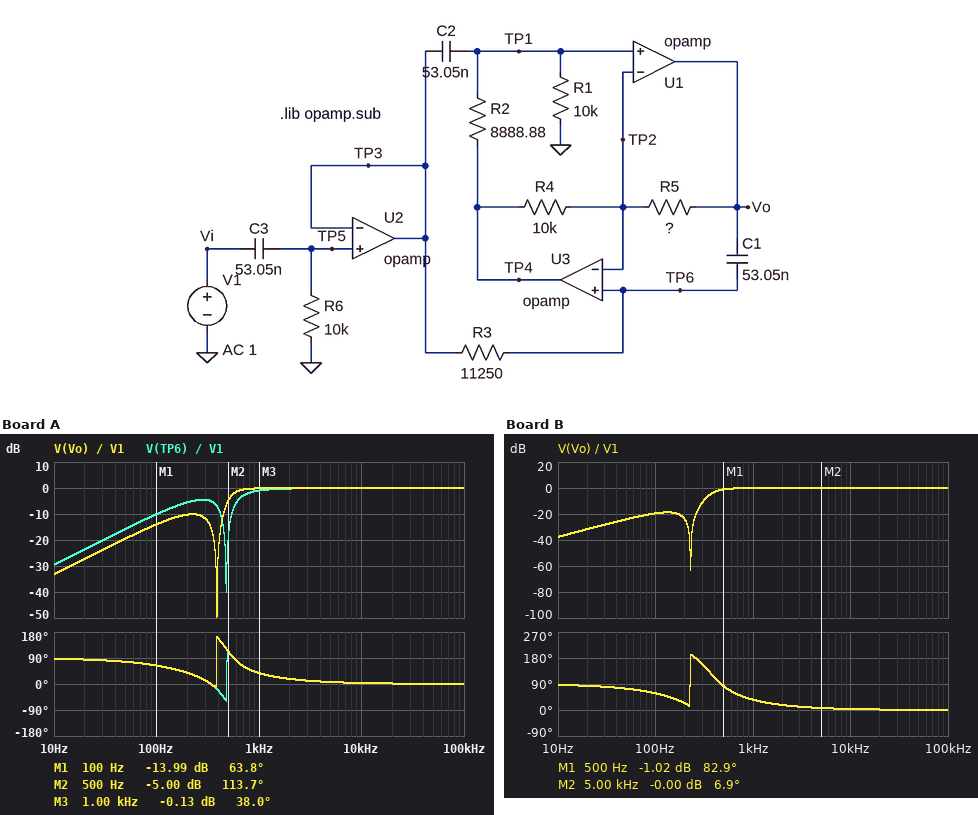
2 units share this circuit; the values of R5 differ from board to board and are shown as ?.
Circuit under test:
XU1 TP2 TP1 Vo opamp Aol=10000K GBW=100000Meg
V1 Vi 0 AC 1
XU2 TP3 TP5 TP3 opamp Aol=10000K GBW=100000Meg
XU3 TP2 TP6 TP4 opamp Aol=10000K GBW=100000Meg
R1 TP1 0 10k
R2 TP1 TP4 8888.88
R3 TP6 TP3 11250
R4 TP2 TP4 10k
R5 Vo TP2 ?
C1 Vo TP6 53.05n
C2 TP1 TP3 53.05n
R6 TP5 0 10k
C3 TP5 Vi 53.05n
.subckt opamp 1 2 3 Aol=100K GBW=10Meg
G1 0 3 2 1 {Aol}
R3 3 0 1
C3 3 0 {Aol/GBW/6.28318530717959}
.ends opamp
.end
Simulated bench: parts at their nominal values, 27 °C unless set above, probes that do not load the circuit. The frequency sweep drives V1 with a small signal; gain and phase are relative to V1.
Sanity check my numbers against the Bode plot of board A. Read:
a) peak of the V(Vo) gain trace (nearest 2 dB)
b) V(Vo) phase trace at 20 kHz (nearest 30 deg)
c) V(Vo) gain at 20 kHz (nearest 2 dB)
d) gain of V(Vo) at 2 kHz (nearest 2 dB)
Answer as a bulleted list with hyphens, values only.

- 0 dB
- 0 deg
- 0 dB
- 0 dB
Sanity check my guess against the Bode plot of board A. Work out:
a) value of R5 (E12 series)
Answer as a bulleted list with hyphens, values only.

- 3.9 kΩ
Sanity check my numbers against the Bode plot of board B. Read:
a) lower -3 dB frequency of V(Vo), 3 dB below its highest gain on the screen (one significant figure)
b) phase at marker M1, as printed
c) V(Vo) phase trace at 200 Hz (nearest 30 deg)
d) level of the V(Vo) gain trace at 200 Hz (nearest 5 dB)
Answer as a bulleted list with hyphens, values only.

- 400 Hz
- 82.9 deg
- 30 deg
- -25 dB
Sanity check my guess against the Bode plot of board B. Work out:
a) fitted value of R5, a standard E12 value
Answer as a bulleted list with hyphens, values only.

- 6.8 kΩ
